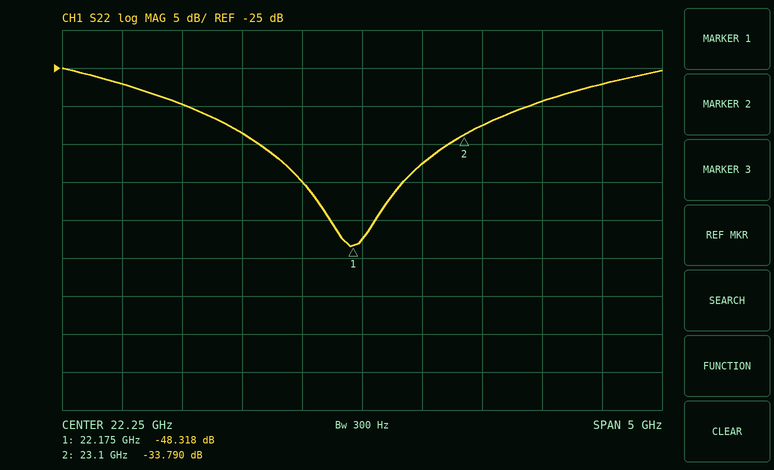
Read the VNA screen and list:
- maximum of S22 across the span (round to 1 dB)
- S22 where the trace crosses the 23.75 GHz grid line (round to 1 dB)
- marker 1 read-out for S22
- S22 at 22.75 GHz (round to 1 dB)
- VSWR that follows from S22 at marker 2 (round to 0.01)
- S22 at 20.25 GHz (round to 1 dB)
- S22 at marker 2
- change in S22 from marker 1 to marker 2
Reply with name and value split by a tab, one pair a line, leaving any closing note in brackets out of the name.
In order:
maximum of S22 across the span	-25 dB
S22 where the trace crosses the 23.75 GHz grid line	-29 dB
marker 1 read-out for S22	-48.318 dB
S22 at 22.75 GHz	-38 dB
VSWR that follows from S22 at marker 2	1.04
S22 at 20.25 GHz	-27 dB
S22 at marker 2	-33.790 dB
change in S22 from marker 1 to marker 2	14.528 dB
